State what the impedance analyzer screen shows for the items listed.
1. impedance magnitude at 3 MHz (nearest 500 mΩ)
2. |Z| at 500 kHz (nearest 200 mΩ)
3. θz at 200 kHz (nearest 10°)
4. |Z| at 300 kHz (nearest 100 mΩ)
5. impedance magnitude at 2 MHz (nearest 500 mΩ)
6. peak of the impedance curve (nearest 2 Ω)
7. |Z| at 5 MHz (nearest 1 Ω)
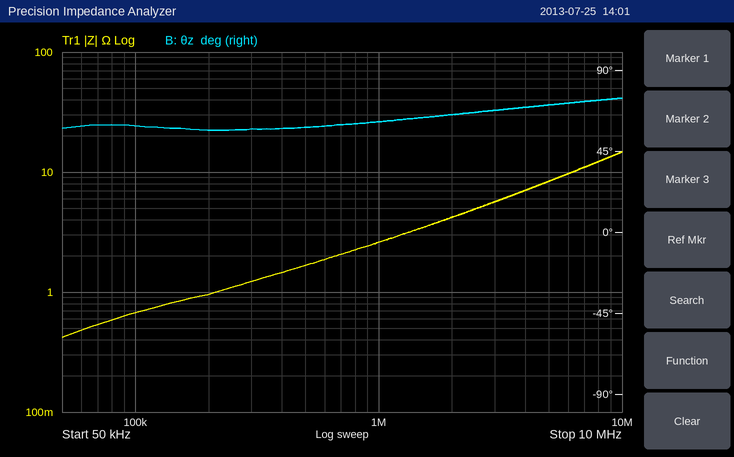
5.5 Ω
1.6 Ω
60°
1.2 Ω
4.0 Ω
14 Ω
8 Ω
